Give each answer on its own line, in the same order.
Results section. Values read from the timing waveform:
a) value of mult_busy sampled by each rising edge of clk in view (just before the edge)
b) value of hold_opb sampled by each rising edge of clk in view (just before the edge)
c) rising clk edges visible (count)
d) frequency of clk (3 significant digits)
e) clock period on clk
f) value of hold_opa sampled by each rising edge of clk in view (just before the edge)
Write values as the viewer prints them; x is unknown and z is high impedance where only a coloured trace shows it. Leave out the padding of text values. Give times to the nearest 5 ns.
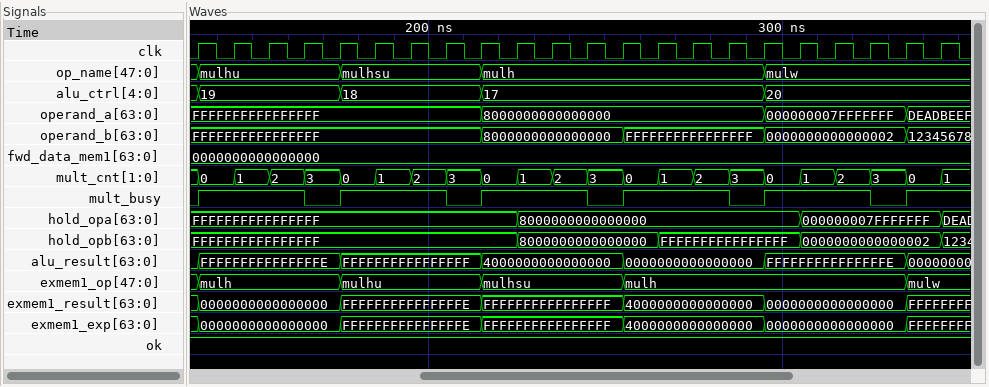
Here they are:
0 1 1 1 0 1 1 1 0 1 1 1 0 1 1 1 0 1 1 1 0 1
FFFFFFFFFFFFFFFF, FFFFFFFFFFFFFFFF, FFFFFFFFFFFFFFFF, FFFFFFFFFFFFFFFF, FFFFFFFFFFFFFFFF, FFFFFFFFFFFFFFFF, FFFFFFFFFFFFFFFF, FFFFFFFFFFFFFFFF, FFFFFFFFFFFFFFFF, FFFFFFFFFFFFFFFF, 8000000000000000, 8000000000000000, 8000000000000000, 8000000000000000, FFFFFFFFFFFFFFFF, FFFFFFFFFFFFFFFF, FFFFFFFFFFFFFFFF, FFFFFFFFFFFFFFFF, 0000000000000002, 0000000000000002, 0000000000000002, 0000000000000002
22
100 MHz
10 ns
FFFFFFFFFFFFFFFF, FFFFFFFFFFFFFFFF, FFFFFFFFFFFFFFFF, FFFFFFFFFFFFFFFF, FFFFFFFFFFFFFFFF, FFFFFFFFFFFFFFFF, FFFFFFFFFFFFFFFF, FFFFFFFFFFFFFFFF, FFFFFFFFFFFFFFFF, FFFFFFFFFFFFFFFF, 8000000000000000, 8000000000000000, 8000000000000000, 8000000000000000, 8000000000000000, 8000000000000000, 8000000000000000, 8000000000000000, 000000007FFFFFFF, 000000007FFFFFFF, 000000007FFFFFFF, 000000007FFFFFFF
